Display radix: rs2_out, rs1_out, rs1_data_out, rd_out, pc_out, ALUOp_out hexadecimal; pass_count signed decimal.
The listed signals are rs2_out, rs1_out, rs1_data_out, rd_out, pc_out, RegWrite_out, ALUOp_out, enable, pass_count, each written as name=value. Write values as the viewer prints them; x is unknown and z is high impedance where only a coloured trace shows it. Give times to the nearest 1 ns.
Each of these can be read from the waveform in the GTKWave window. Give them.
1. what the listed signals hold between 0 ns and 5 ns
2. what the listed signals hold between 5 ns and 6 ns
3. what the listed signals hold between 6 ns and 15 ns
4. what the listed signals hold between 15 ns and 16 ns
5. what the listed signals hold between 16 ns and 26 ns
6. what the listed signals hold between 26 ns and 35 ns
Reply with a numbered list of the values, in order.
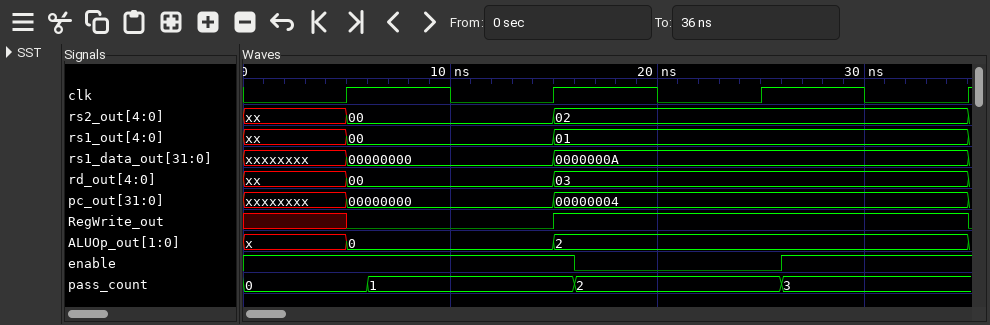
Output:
1. rs2_out=xx, rs1_out=xx, rs1_data_out=xxxxxxxx, rd_out=xx, pc_out=xxxxxxxx, RegWrite_out=x, ALUOp_out=x, enable=1, pass_count=0
2. rs2_out=00, rs1_out=00, rs1_data_out=00000000, rd_out=00, pc_out=00000000, RegWrite_out=0, ALUOp_out=0, enable=1, pass_count=0
3. rs2_out=00, rs1_out=00, rs1_data_out=00000000, rd_out=00, pc_out=00000000, RegWrite_out=0, ALUOp_out=0, enable=1, pass_count=1
4. rs2_out=02, rs1_out=01, rs1_data_out=0000000A, rd_out=03, pc_out=00000004, RegWrite_out=1, ALUOp_out=2, enable=1, pass_count=1
5. rs2_out=02, rs1_out=01, rs1_data_out=0000000A, rd_out=03, pc_out=00000004, RegWrite_out=1, ALUOp_out=2, enable=0, pass_count=2
6. rs2_out=02, rs1_out=01, rs1_data_out=0000000A, rd_out=03, pc_out=00000004, RegWrite_out=1, ALUOp_out=2, enable=1, pass_count=3
